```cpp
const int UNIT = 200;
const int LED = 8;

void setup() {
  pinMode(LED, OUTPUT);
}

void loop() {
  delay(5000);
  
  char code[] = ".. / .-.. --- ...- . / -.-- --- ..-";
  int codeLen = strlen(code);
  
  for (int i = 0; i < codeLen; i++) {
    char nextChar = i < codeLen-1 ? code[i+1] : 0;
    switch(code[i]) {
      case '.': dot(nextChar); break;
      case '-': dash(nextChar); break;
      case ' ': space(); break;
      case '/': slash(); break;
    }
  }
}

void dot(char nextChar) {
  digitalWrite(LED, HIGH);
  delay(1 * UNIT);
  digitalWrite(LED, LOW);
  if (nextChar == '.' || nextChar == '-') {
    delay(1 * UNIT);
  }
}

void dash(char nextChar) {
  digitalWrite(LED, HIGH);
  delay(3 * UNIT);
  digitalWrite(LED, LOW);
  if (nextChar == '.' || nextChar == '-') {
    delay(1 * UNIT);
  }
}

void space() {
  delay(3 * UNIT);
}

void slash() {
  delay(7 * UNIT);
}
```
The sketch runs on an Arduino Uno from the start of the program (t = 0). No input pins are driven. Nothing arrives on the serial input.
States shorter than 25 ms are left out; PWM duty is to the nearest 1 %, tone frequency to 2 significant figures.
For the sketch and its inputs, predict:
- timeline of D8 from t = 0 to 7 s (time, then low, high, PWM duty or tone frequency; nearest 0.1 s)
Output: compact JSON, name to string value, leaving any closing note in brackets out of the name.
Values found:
{"timeline of D8 from t = 0 to 7 s": "0 s low; 5 s high; 5.2 s low; 5.4 s high; 5.6 s low"}
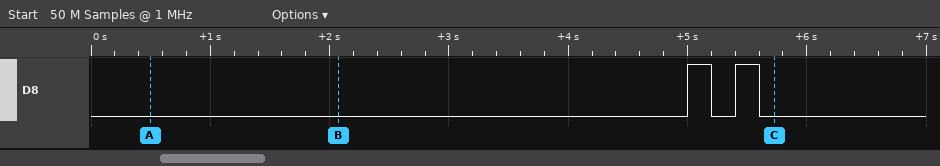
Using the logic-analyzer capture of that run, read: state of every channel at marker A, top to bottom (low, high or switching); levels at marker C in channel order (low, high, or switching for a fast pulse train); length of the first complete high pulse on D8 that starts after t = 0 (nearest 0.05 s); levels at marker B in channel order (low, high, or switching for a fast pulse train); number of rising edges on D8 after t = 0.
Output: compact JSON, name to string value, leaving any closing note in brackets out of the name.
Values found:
{"state of every channel at marker A, top to bottom": "D8 low", "levels at marker C in channel order": "D8 low", "length of the first complete high pulse on D8 that starts after t = 0": "0.20 s", "levels at marker B in channel order": "D8 low", "number of rising edges on D8 after t = 0": "2"}
